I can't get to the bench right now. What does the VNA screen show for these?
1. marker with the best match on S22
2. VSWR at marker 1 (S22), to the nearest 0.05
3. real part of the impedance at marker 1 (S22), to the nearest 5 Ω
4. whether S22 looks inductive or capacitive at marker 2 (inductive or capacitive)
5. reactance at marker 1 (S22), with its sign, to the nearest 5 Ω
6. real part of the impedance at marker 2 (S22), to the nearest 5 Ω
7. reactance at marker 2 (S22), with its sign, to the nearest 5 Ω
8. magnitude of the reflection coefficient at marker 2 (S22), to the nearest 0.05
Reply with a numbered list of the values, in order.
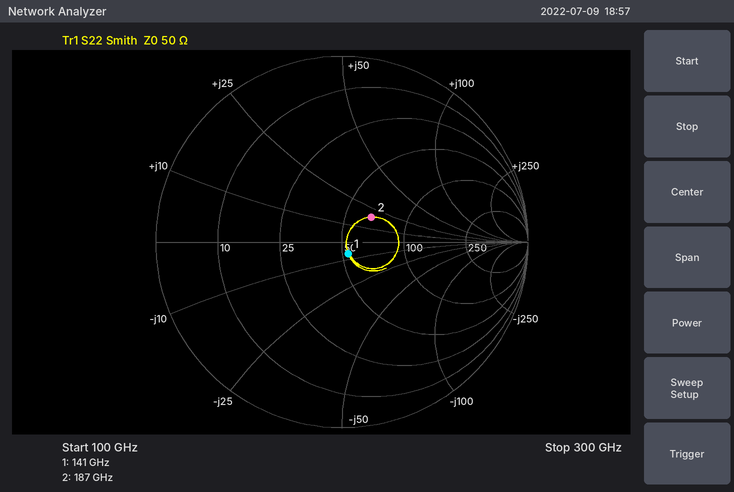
1. marker 1
2. 1.15
3. 55 Ω
4. inductive
5. -5 Ω
6. 65 Ω
7. +20 Ω
8. 0.20
